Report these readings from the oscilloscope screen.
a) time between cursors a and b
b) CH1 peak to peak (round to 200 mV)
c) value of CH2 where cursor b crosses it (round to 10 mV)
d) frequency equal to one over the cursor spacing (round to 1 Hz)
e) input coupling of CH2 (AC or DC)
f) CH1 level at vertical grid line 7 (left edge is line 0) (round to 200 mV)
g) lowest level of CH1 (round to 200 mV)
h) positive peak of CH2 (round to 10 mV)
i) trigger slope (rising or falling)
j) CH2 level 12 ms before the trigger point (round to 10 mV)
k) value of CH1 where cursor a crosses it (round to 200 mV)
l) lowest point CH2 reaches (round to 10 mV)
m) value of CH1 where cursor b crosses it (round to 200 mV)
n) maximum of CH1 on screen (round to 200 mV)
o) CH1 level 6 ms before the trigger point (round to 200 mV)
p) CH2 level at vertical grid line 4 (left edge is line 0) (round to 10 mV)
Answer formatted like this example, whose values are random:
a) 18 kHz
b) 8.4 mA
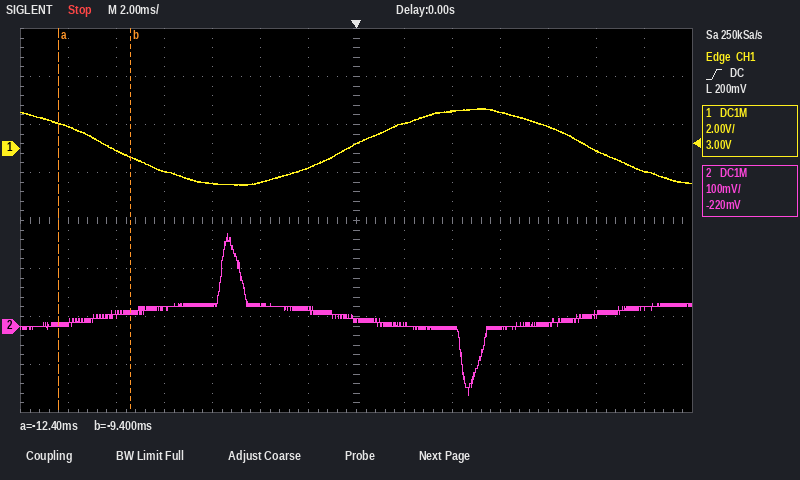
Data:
a) 3.0 ms
b) 3.2 V
c) 30 mV
d) 333 Hz
e) DC
f) 200 mV
g) -1.6 V
h) 190 mV
i) rising
j) 10 mV
k) 1.0 V
l) -140 mV
m) -400 mV
n) 1.6 V
o) -1.4 V
p) 40 mV
